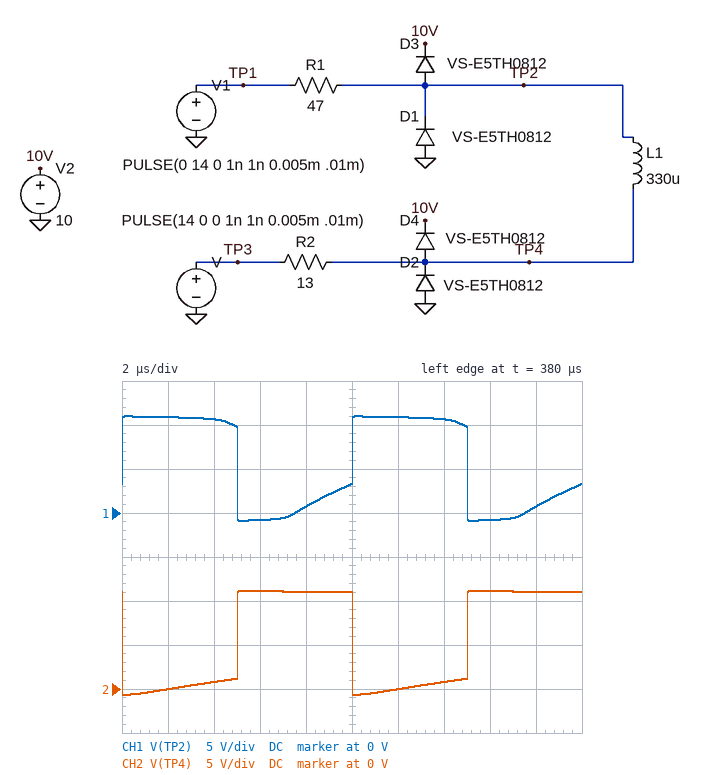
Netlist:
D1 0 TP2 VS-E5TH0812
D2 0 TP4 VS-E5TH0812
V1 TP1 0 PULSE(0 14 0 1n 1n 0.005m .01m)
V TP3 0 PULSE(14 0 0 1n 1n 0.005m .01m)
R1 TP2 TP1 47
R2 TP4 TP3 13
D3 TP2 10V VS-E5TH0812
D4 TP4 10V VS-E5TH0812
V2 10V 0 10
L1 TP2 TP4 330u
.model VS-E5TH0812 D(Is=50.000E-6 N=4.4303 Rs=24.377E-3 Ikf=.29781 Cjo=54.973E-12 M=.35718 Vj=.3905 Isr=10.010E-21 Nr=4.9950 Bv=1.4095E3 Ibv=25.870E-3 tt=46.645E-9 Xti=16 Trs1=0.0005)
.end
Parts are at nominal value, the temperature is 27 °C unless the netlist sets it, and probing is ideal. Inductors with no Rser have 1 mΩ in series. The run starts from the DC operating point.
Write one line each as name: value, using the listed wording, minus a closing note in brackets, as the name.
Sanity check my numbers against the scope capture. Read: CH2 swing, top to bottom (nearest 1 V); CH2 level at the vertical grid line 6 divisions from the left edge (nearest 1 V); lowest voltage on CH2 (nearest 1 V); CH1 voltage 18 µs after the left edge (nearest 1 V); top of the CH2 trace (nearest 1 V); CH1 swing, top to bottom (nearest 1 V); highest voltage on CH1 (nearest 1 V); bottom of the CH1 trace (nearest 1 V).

CH2 swing, top to bottom: 12 V
CH2 level at the vertical grid line 6 divisions from the left edge: 0 V
lowest voltage on CH2: -1 V
CH1 voltage 18 µs after the left edge: 1 V
top of the CH2 trace: 11 V
CH1 swing, top to bottom: 12 V
highest voltage on CH1: 11 V
bottom of the CH1 trace: -1 V
